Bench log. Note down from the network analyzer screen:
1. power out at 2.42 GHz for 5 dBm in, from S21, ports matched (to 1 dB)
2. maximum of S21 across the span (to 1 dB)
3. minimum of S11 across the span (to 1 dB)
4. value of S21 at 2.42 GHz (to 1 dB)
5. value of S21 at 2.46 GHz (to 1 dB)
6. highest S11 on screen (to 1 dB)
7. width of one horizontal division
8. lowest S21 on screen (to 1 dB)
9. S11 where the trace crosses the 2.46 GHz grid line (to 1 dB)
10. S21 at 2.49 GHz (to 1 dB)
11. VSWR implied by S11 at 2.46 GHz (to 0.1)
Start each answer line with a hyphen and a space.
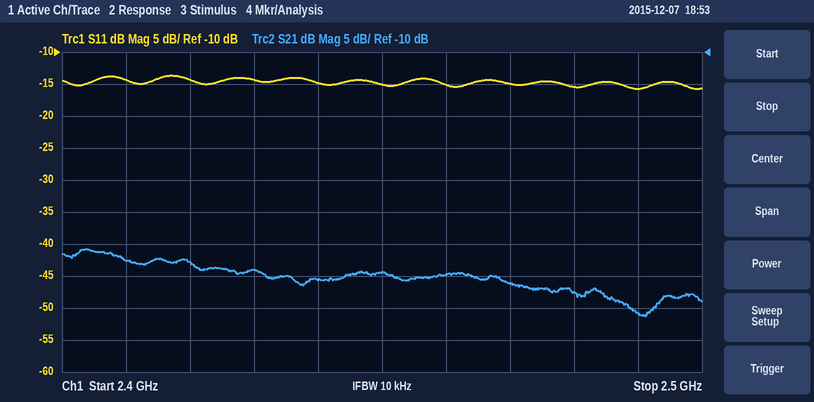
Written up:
- -38 dBm
- -41 dB
- -16 dB
- -43 dB
- -45 dB
- -14 dB
- 10 MHz
- -51 dB
- -15 dB
- -51 dB
- 1.4
